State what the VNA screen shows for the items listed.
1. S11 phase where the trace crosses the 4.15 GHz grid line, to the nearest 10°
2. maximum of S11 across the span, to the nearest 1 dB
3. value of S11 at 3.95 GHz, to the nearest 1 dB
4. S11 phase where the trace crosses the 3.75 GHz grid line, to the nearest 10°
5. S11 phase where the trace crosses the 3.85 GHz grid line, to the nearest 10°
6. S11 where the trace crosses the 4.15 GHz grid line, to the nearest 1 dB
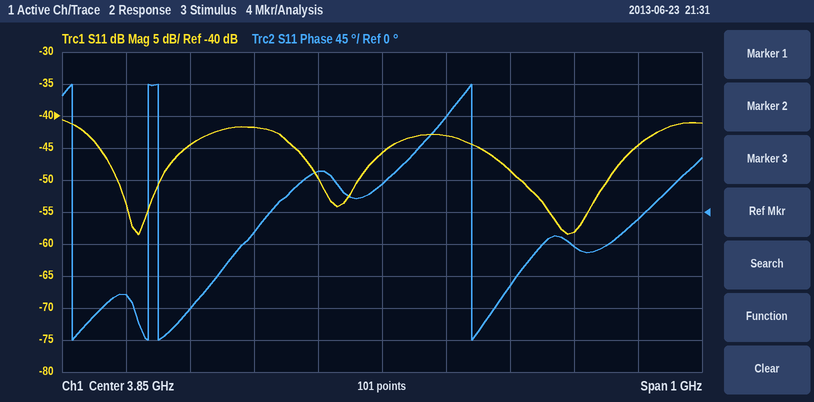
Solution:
-50°
-41 dB
-43 dB
60°
40°
-58 dB
